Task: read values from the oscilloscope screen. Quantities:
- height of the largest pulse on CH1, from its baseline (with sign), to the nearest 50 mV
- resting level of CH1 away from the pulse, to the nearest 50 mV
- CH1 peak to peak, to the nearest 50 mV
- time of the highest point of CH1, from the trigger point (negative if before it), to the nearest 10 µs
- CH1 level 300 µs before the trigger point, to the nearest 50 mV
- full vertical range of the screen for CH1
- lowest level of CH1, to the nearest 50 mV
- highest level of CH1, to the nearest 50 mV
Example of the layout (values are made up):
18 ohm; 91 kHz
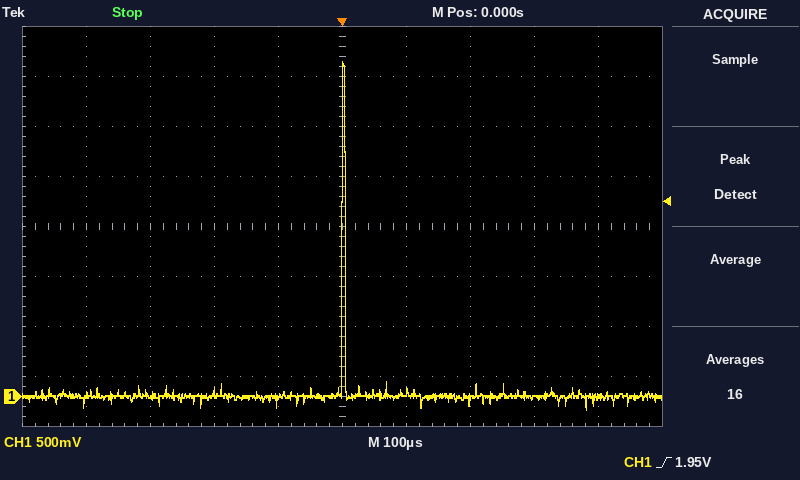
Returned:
+3.35 V; 0 mV; 3.50 V; 0 µs; 0 mV; 4 V; -150 mV; 3.35 V
